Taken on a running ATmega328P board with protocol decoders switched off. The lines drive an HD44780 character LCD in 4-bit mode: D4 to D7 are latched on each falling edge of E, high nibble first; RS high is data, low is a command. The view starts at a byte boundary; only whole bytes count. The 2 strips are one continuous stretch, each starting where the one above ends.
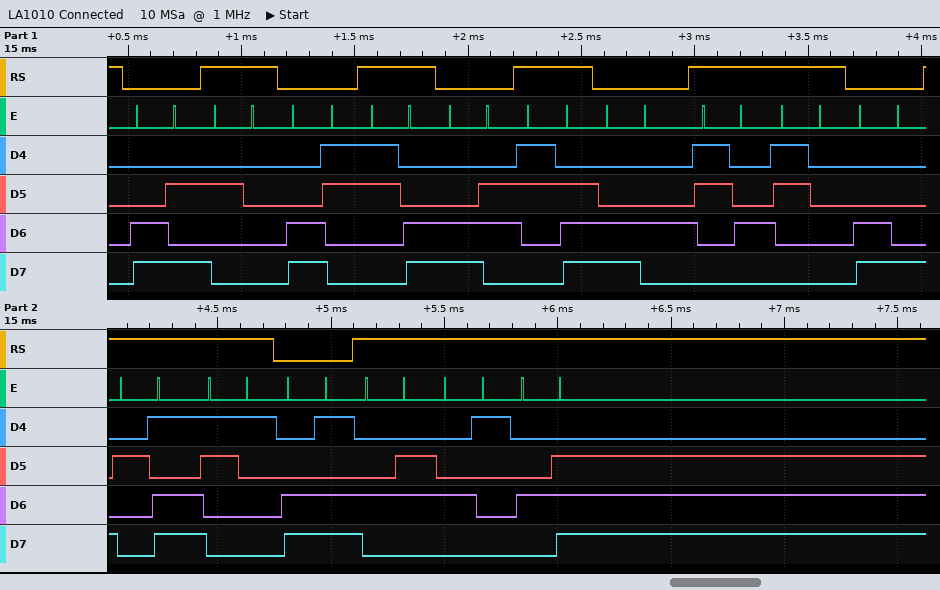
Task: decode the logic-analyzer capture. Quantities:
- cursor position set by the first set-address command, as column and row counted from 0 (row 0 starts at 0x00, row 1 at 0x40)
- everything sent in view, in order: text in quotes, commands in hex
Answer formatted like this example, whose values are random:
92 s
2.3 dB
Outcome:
column 10, row 1
0xCA " " 0xC3 "<" 0xC6 ">" 0xC4 "40" 0xC8 "-1" 0xCD "FAN"
